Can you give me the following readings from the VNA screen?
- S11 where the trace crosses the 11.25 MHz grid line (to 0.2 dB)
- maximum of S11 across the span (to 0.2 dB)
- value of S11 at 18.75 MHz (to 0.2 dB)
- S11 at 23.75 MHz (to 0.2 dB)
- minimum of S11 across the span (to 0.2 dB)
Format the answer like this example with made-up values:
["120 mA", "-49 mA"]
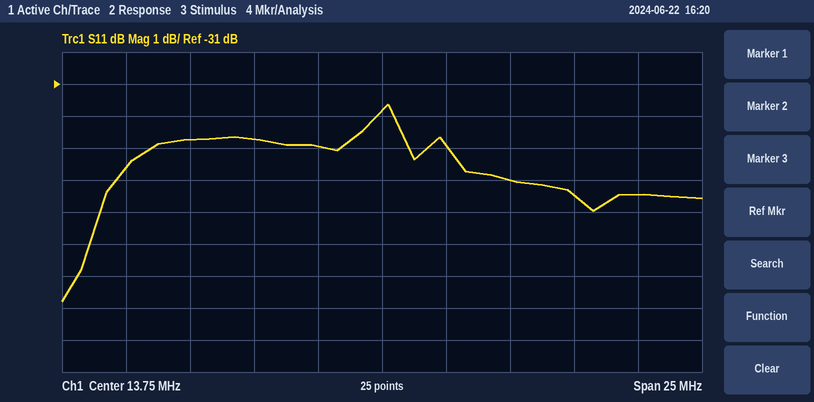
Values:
["-33.0 dB", "-31.6 dB", "-34.0 dB", "-34.4 dB", "-37.8 dB"]
